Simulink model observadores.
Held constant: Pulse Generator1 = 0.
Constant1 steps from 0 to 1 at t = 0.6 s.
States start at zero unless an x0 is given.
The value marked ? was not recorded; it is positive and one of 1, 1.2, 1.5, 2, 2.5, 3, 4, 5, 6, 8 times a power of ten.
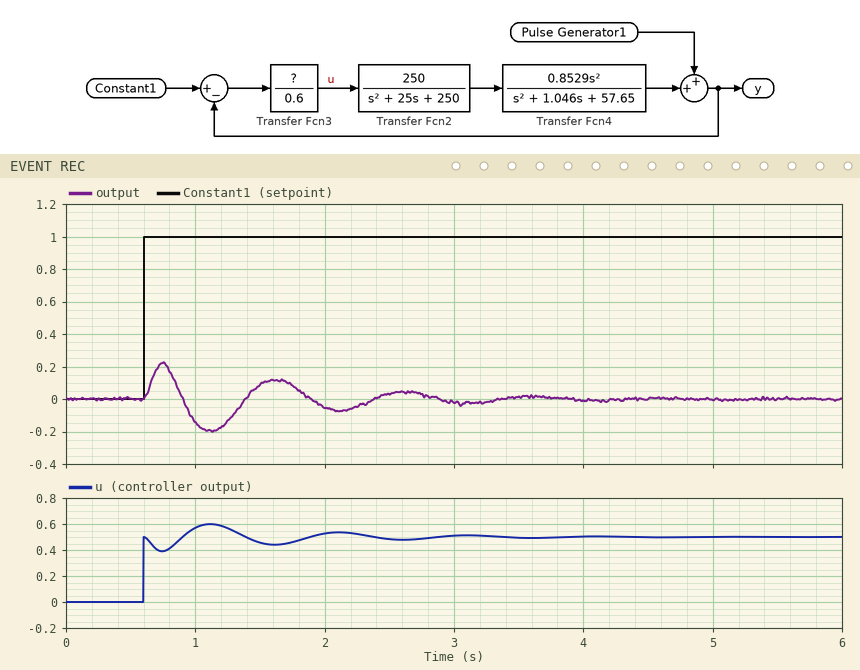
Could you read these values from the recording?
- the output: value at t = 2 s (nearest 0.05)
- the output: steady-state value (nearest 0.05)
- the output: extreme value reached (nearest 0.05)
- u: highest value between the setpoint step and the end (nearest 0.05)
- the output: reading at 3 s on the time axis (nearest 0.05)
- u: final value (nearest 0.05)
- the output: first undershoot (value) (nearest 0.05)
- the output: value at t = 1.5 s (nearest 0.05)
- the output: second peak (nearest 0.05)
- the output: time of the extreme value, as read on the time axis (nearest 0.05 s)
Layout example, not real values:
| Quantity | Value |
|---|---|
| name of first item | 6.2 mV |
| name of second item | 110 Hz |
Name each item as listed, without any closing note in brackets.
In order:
| Quantity | Value |
|---|---|
| the output: value at t = 2 s | -0.05 |
| the output: steady-state value | 0.00 |
| the output: extreme value reached | 0.20 |
| u: highest value between the setpoint step and the end | 0.60 |
| the output: reading at 3 s on the time axis | 0.00 |
| u: final value | 0.50 |
| the output: first undershoot (value) | -0.20 |
| the output: value at t = 1.5 s | 0.10 |
| the output: second peak | 0.10 |
| the output: time of the extreme value, as read on the time axis | 0.75 s |
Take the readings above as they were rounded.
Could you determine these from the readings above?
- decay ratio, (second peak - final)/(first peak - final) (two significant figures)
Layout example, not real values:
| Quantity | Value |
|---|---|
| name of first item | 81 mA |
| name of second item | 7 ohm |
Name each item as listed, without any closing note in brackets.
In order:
| Quantity | Value |
|---|---|
| decay ratio, (second peak - final)/(first peak - final) | 0.50 |
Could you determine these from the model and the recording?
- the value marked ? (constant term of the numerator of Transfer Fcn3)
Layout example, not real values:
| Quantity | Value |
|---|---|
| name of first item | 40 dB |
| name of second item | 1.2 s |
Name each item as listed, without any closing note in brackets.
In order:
| Quantity | Value |
|---|---|
| the value marked ? | 0.3 |
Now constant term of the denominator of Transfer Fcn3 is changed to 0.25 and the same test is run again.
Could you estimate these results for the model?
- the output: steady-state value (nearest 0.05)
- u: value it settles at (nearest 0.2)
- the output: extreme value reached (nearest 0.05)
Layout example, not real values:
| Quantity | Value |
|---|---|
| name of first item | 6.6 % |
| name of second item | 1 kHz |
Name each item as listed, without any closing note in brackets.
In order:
| Quantity | Value |
|---|---|
| the output: steady-state value | 0.00 |
| u: value it settles at | 1.2 |
| the output: extreme value reached | 0.45 |
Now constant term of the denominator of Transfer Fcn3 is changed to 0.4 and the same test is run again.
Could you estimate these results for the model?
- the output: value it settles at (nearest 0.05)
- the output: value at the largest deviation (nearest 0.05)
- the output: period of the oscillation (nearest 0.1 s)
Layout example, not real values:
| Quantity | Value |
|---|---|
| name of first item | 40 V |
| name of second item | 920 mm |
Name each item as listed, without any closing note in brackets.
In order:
| Quantity | Value |
|---|---|
| the output: value it settles at | 0.00 |
| the output: value at the largest deviation | 0.30 |
| the output: period of the oscillation | 0.9 s |
